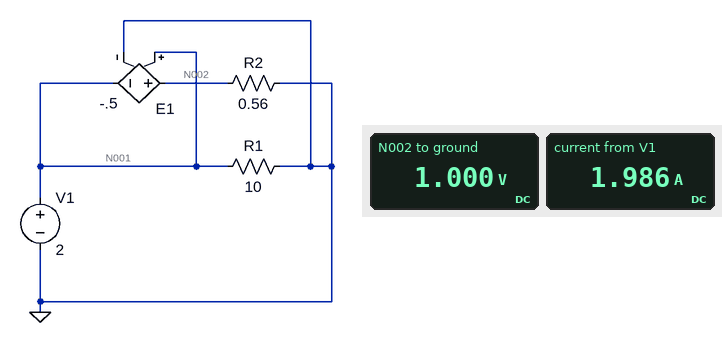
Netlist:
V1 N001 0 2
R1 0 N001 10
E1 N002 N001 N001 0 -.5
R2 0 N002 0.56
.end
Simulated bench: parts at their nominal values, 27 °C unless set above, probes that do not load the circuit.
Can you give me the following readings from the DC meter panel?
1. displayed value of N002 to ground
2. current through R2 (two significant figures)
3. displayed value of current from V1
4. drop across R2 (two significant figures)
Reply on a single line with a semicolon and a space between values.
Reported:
1.000 V; 1.8 A; 1.986 A; 1.0 V
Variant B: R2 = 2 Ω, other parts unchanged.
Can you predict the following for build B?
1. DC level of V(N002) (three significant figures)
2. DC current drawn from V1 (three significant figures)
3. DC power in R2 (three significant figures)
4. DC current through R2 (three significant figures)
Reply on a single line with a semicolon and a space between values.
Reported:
1.00 V; 700 mA; 500 mW; 500 mA
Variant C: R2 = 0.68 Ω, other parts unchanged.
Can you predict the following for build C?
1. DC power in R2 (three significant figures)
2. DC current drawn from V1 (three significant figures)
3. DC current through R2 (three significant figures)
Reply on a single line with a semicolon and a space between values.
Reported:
1.47 W; 1.67 A; 1.47 A
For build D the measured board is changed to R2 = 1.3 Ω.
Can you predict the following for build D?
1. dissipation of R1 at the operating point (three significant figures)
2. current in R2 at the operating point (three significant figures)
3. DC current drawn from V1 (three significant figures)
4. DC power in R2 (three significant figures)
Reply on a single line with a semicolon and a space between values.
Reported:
400 mW; 769 mA; 969 mA; 769 mW
